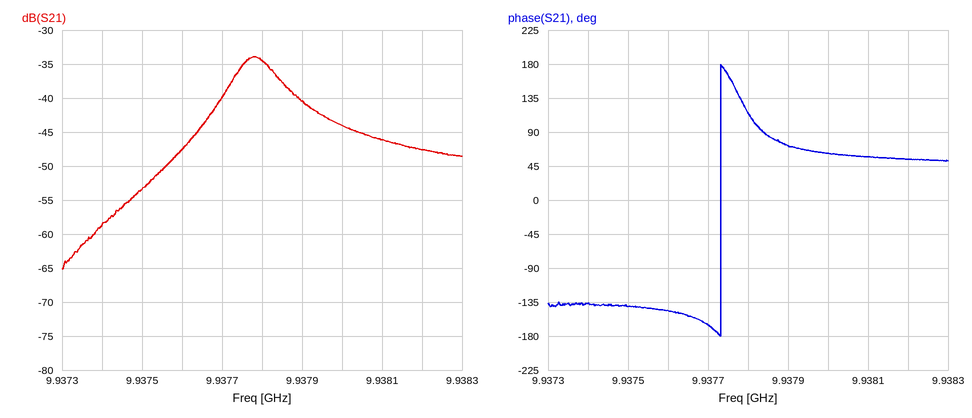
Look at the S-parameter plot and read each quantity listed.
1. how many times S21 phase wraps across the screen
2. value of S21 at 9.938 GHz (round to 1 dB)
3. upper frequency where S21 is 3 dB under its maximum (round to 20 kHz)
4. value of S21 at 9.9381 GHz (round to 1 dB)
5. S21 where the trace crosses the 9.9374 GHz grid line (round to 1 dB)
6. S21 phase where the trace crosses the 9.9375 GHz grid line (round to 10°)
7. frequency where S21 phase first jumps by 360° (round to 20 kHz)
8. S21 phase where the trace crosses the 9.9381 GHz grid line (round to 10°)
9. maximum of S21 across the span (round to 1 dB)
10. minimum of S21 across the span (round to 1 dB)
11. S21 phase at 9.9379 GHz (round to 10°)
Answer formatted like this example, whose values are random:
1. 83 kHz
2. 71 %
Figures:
1. 1
2. -44 dB
3. 9.93784 GHz
4. -46 dB
5. -59 dB
6. -140°
7. 9.93774 GHz
8. 60°
9. -34 dB
10. -65 dB
11. 70°
